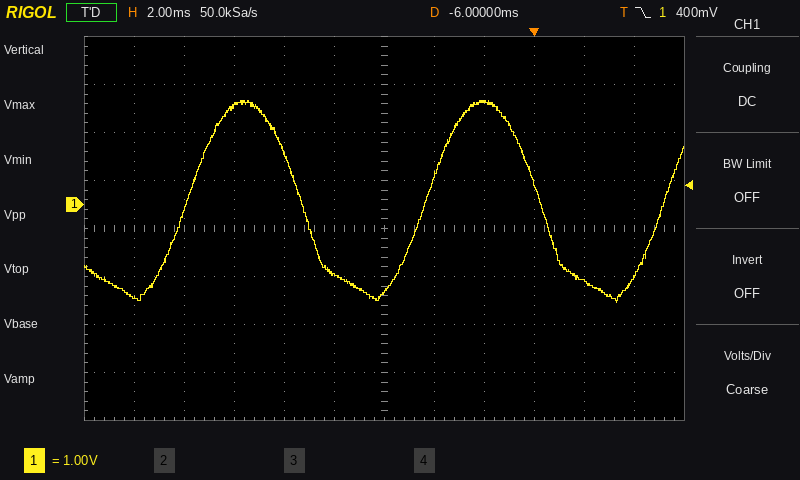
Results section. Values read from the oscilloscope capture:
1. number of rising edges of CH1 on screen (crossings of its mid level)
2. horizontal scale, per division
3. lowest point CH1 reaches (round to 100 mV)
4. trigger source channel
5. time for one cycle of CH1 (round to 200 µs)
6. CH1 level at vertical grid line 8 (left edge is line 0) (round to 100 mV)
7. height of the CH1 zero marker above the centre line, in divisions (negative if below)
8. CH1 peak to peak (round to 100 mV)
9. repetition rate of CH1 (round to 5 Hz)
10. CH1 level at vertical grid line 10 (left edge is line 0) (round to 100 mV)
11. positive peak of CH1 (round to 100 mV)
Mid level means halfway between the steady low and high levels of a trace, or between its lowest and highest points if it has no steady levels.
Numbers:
3
2 ms
-2.0 V
CH1
9.6 ms
2.1 V
+0.5 div
4.2 V
105 Hz
-1.6 V
2.2 V
